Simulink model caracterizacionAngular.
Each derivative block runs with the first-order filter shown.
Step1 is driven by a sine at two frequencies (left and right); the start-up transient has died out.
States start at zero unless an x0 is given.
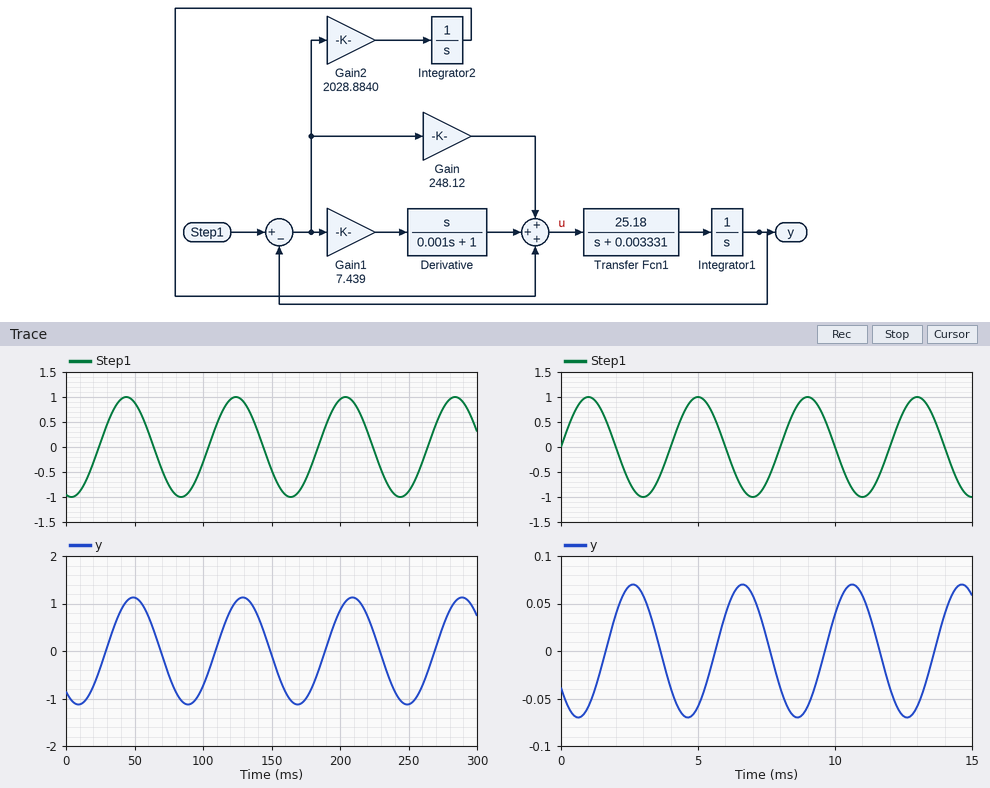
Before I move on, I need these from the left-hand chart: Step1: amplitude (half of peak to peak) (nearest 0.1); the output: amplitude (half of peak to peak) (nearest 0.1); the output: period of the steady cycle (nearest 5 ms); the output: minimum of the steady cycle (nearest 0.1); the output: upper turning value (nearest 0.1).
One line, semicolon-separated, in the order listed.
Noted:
1.0; 1.1; 80 ms; -1.1; 1.1
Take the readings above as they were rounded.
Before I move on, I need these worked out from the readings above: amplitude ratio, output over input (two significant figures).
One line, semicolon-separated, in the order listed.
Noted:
1.1
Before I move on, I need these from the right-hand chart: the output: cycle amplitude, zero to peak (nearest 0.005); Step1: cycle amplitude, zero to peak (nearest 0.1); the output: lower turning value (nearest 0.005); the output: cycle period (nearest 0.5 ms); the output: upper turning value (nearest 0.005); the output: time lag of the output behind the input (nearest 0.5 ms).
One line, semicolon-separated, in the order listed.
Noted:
0.070; 1.0; -0.070; 4.0 ms; 0.070; 1.5 ms
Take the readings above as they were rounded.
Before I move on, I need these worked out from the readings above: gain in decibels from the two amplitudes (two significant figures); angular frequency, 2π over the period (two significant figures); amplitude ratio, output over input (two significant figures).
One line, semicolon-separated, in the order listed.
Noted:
-23 dB; 1.6 rad/ms; 0.070
